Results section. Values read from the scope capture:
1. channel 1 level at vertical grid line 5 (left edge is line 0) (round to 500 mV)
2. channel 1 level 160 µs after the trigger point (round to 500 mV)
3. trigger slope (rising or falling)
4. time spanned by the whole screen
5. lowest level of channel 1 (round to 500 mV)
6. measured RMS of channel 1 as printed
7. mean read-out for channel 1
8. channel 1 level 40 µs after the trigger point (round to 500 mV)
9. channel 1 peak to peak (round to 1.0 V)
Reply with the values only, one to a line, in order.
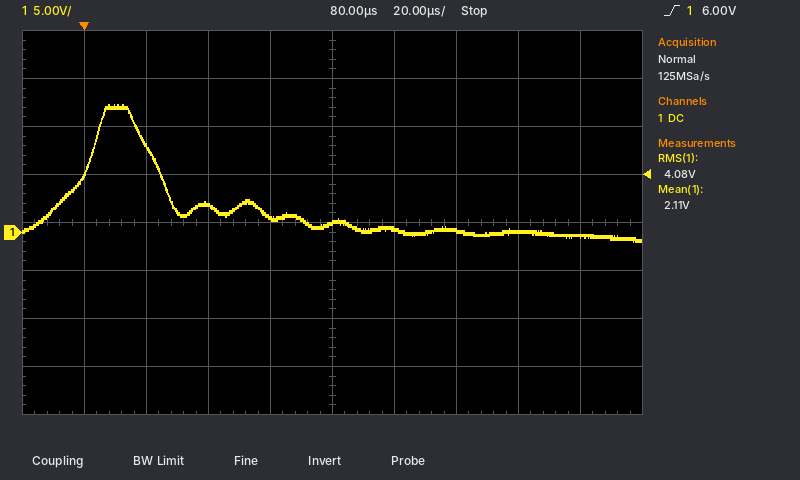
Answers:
1.0 V
-500 mV
rising
200 µs
-1.0 V
4.08 V
2.11 V
3.0 V
14.0 V
